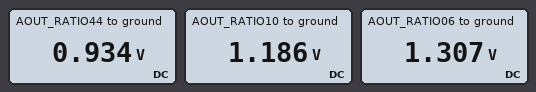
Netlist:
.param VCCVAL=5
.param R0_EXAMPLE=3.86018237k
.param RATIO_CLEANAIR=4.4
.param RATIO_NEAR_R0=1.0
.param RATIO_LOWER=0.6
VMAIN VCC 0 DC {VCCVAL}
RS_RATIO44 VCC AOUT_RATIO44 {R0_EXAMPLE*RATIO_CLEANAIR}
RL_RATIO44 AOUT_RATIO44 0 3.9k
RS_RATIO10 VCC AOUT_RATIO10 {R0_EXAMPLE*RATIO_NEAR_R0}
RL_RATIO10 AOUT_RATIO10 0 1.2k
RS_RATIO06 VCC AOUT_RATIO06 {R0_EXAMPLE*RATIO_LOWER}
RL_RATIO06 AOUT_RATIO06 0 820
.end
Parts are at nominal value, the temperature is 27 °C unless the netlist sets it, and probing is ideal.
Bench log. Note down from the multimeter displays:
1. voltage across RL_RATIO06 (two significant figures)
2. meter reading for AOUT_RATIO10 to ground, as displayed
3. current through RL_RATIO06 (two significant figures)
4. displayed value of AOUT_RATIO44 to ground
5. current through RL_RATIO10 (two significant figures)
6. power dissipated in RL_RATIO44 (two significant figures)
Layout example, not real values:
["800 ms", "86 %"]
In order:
["1.3 V", "1.186 V", "1.6 mA", "0.934 V", "990 µA", "220 µW"]
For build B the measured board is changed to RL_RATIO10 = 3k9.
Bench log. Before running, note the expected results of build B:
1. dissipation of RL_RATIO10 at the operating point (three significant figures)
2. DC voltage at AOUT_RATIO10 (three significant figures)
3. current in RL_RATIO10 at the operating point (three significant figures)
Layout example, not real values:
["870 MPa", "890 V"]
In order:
["1.62 mW", "2.51 V", "644 µA"]
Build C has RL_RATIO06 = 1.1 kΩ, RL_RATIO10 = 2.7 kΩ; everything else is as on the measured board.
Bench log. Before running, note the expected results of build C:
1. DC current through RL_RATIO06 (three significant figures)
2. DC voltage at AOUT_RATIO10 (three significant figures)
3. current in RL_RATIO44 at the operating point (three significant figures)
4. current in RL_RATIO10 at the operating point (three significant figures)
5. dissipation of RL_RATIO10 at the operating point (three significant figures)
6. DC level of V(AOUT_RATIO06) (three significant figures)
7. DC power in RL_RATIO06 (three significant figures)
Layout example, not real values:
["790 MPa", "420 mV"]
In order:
["1.46 mA", "2.06 V", "239 µA", "762 µA", "1.57 mW", "1.61 V", "2.36 mW"]
